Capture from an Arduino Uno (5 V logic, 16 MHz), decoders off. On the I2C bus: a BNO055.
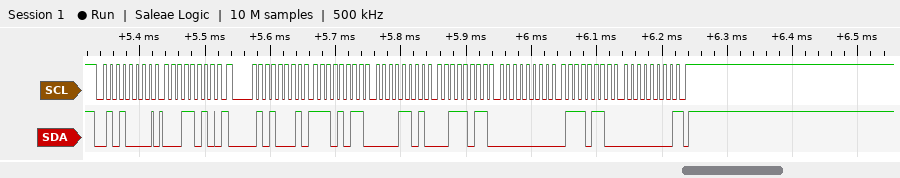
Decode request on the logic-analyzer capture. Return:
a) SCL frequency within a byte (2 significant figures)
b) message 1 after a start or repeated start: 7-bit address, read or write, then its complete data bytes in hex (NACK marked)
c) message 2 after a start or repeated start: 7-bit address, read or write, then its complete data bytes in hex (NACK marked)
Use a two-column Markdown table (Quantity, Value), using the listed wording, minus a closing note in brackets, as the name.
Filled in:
| Quantity | Value |
|---|---|
| SCL frequency within a byte | 100 kHz |
| message 1 after a start or repeated start: 7-bit address, read or write, then its complete data bytes in hex | 0x28 write: 1A |
| message 2 after a start or repeated start: 7-bit address, read or write, then its complete data bytes in hex | 0x28 read: EB 0D 3B 00 76 00 NACK |
